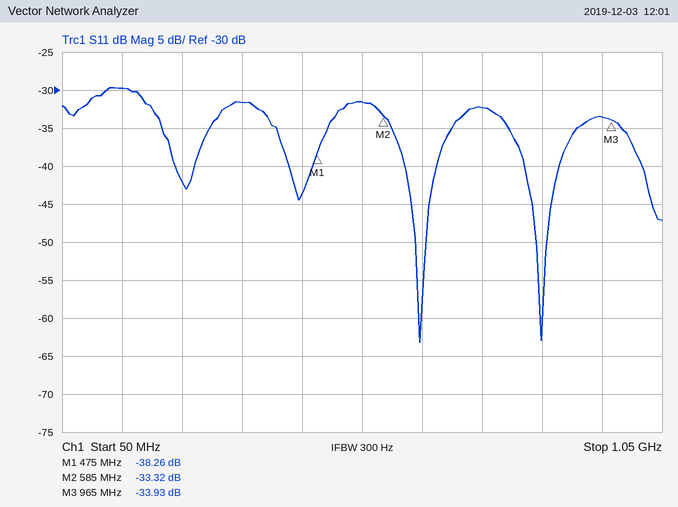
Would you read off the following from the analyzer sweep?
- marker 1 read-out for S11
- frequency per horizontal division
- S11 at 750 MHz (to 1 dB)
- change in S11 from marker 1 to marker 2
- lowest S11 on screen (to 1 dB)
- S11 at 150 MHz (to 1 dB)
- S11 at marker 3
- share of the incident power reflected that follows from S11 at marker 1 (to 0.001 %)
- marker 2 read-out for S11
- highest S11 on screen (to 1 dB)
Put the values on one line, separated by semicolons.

-38.26 dB; 100 MHz; -32 dB; 4.94 dB; -63 dB; -30 dB; -33.93 dB; 0.015 %; -33.32 dB; -30 dB
